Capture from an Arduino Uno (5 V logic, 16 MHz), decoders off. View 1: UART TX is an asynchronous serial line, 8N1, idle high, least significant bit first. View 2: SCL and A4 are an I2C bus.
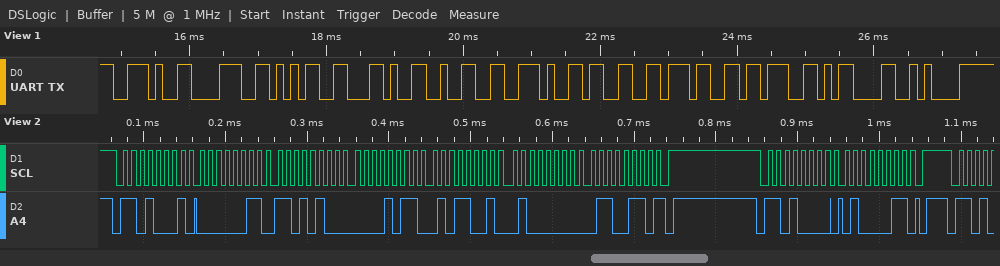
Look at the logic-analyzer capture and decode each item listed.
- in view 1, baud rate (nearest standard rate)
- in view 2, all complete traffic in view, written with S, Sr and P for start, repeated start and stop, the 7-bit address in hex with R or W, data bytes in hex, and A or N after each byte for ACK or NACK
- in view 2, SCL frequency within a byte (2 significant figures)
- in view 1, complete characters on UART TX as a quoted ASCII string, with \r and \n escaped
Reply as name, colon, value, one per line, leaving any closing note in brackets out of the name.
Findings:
in view 1, baud rate: 9600 baud
in view 2, all complete traffic in view, written with S, Sr and P for start, repeated start and stop, the 7-bit address in hex with R or W, data bytes in hex, and A or N after each byte for ACK or NACK: S 68R A 03 A D4 A 0B A 59 A 40 A 66 N P S 68W A 43 A P
in view 2, SCL frequency within a byte: 100 kHz
in view 1, complete characters on UART TX as a quoted ASCII string, with \r and \n escaped: ".85,2.37;\r\n"
